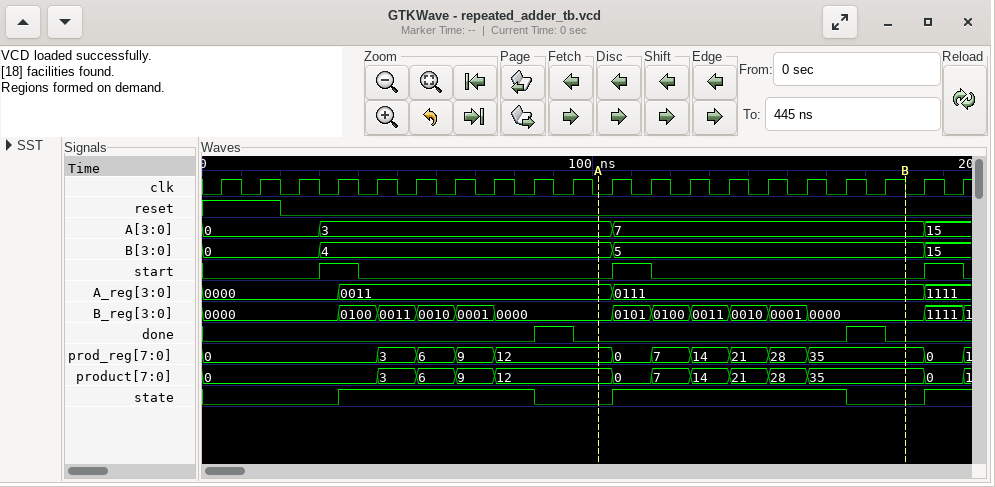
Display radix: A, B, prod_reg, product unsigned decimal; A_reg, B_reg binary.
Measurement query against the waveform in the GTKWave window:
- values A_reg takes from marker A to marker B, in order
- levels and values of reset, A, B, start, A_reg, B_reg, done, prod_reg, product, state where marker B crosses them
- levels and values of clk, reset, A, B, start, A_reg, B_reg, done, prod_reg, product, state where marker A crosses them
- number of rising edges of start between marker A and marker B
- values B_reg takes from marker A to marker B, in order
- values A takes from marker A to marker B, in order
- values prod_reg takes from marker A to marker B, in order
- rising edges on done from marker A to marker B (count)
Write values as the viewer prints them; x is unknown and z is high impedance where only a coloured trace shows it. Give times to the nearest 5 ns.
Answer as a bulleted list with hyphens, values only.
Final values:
- 0011, 0111
- reset=0, A=7, B=5, start=0, A_reg=0111, B_reg=0000, done=0, prod_reg=35, product=35, state=0
- clk=0, reset=0, A=3, B=4, start=0, A_reg=0011, B_reg=0000, done=0, prod_reg=12, product=12, state=0
- 1
- 0000, 0101, 0100, 0011, 0010, 0001, 0000
- 3, 7
- 12, 0, 7, 14, 21, 28, 35
- 1
